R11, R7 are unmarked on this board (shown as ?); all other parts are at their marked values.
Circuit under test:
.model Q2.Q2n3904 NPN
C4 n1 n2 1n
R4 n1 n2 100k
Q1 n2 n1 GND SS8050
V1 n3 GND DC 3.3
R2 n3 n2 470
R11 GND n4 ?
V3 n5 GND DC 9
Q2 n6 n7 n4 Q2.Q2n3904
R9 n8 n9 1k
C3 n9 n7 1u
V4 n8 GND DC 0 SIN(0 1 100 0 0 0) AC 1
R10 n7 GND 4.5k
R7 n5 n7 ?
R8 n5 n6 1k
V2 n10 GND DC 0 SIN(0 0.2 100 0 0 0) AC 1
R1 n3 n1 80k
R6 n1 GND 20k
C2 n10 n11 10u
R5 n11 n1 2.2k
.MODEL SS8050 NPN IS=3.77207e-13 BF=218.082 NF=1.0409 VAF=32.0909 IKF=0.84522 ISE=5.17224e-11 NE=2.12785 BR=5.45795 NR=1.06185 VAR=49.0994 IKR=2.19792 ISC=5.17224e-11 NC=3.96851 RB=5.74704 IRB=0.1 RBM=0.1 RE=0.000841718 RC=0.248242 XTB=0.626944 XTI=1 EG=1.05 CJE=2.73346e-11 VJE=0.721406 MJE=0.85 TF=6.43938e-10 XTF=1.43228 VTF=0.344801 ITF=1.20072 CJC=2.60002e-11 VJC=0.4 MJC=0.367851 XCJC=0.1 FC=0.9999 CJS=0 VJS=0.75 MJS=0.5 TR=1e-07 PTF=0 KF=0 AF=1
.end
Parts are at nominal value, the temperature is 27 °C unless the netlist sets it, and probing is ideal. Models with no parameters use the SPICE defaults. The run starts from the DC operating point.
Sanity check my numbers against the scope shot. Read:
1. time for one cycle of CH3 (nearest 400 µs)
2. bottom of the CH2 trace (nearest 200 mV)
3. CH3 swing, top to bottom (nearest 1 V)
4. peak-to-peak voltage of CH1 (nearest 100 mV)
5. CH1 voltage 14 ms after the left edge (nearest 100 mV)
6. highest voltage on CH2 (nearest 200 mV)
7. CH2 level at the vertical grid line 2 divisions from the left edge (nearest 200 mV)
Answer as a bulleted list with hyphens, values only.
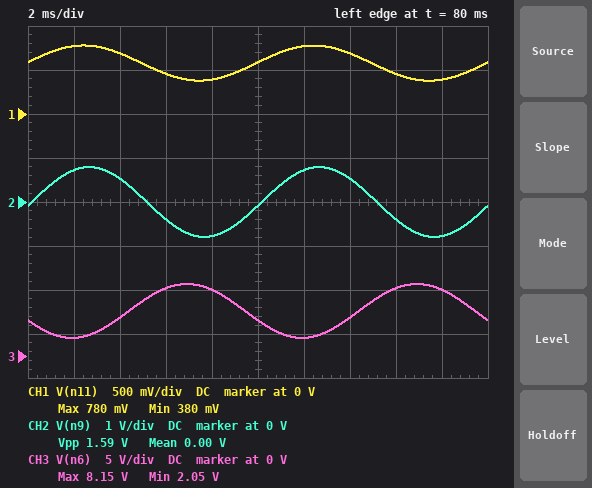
- 10.0 ms
- -800 mV
- 6 V
- 400 mV
- 700 mV
- 800 mV
- 600 mV
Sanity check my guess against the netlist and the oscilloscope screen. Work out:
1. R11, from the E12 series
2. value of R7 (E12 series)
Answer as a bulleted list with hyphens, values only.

- 220 Ω
- 18 kΩ
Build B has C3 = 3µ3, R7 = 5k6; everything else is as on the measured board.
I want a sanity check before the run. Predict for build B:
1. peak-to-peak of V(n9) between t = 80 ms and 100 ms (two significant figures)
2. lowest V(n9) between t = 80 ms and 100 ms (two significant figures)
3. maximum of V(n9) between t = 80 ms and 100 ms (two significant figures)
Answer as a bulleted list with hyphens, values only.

- 790 mV
- -370 mV
- 420 mV
